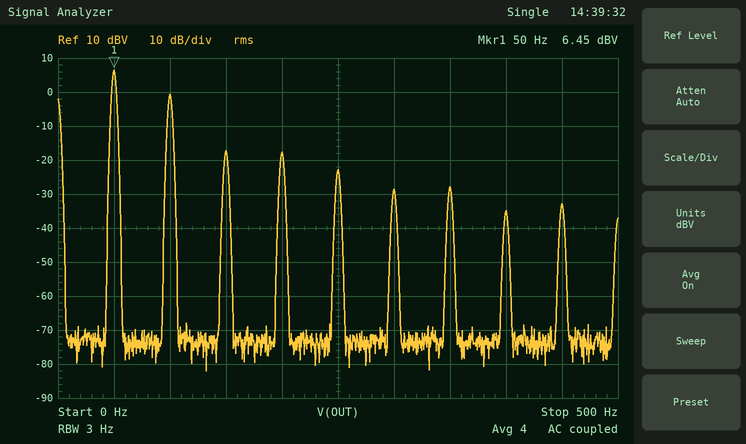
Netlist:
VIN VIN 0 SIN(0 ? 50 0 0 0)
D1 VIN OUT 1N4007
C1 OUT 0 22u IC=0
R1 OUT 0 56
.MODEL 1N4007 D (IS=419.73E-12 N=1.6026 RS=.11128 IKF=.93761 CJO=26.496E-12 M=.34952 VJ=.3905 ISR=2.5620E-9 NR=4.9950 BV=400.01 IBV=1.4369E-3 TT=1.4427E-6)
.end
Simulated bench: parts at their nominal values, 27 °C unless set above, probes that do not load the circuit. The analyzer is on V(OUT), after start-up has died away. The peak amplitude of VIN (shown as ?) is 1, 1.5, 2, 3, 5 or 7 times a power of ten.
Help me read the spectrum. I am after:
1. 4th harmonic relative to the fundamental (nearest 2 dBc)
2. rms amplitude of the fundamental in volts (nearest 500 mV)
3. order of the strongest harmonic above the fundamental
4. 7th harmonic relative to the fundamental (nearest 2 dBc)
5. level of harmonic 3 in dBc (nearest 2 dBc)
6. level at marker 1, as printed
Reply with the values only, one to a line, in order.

-24 dBc
2.0 V
2
-34 dBc
-24 dBc
6.45 dBV
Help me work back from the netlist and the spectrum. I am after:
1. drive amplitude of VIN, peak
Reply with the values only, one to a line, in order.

7 V
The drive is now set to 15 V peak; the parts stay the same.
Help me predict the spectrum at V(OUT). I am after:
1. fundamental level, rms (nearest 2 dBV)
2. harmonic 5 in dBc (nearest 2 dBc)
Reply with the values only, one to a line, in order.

14 dBV
-32 dBc
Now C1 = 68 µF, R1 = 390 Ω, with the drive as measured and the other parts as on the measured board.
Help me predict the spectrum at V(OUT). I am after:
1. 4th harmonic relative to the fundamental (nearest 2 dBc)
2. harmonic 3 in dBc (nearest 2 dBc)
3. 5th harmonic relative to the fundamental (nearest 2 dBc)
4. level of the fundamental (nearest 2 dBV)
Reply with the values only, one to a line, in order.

-16 dBc
-12 dBc
-22 dBc
-2 dBV
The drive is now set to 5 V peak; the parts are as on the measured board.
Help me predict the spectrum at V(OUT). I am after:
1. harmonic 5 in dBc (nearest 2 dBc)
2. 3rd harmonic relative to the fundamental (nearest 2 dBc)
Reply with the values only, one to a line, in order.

-28 dBc
-22 dBc
